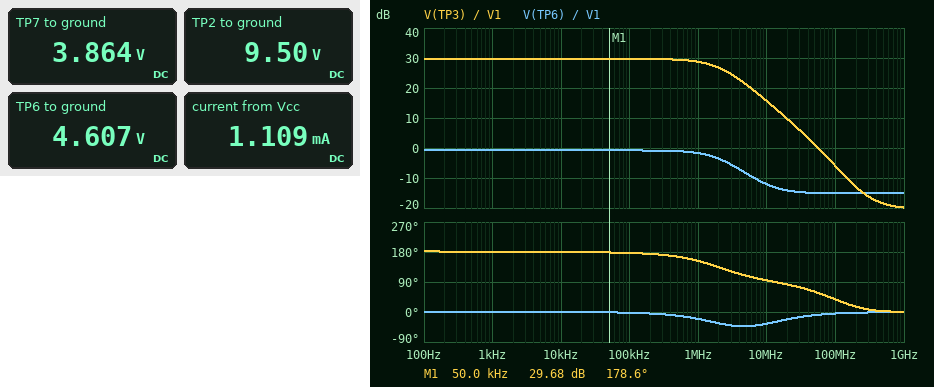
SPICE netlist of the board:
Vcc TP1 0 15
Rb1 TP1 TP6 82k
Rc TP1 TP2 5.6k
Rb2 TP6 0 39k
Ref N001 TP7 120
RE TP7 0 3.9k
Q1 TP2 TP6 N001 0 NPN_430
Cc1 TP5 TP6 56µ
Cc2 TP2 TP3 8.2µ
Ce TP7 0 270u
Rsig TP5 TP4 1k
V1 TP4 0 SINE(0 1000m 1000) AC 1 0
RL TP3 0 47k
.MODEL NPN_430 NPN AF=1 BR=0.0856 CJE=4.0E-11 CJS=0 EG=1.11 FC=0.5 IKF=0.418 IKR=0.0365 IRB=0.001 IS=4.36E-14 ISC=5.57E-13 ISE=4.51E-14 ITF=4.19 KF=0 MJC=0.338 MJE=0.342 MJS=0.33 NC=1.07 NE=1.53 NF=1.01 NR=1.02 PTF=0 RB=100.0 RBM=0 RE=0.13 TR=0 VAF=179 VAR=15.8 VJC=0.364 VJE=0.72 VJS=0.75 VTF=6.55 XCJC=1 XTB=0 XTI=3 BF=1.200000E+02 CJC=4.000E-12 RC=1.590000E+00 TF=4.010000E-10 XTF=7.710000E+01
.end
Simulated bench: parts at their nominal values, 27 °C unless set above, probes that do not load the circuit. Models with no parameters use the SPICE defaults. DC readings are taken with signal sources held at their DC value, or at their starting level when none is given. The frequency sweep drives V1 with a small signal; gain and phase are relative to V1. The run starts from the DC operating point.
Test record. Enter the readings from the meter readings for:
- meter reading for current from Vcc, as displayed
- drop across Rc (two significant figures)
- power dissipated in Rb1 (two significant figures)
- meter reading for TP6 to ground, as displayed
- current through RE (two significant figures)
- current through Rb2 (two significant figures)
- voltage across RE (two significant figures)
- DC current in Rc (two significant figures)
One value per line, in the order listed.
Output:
1.109 mA
5.5 V
1.3 mW
4.607 V
990 µA
120 µA
3.9 V
980 µA
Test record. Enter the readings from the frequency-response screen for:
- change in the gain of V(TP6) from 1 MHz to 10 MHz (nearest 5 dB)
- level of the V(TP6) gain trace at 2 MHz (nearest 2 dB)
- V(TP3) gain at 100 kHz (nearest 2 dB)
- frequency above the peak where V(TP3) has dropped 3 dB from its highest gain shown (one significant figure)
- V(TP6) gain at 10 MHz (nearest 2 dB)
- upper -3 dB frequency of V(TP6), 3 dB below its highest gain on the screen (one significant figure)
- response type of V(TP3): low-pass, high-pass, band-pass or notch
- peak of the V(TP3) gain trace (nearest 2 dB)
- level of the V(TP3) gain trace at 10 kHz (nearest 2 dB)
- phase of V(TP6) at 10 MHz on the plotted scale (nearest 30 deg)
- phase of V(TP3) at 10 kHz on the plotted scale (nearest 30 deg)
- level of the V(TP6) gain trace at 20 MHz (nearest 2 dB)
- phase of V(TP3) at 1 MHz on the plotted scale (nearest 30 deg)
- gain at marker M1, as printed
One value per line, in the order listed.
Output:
-10 dB
-4 dB
30 dB
2 MHz
-12 dB
2 MHz
low-pass
30 dB
30 dB
-30 deg
180 deg
-14 dB
150 deg
29.68 dB
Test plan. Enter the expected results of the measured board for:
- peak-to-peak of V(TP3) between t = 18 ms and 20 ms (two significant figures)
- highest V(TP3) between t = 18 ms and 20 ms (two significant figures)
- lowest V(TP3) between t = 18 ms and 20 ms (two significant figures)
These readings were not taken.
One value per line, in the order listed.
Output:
10 V
4.9 V
-5.2 V
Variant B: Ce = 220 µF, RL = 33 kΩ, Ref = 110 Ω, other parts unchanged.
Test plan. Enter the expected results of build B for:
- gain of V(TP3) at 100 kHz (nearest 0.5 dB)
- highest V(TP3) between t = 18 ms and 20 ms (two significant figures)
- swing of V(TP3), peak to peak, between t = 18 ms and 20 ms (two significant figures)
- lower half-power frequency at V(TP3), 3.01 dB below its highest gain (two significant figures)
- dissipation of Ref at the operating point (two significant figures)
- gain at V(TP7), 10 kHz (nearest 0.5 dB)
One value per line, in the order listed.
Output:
30.0 dB
4.7 V
9.9 V
5.3 Hz
110 µW
-66.5 dB
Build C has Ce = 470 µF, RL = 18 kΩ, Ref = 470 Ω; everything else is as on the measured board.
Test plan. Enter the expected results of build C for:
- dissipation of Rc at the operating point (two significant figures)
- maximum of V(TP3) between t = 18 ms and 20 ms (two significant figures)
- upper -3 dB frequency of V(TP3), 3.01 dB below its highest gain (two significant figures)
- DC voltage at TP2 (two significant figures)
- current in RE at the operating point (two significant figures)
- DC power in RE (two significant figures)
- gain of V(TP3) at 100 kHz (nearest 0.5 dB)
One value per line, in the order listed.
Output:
4.6 mW
3.9 V
5.8 MHz
9.9 V
920 µA
3.3 mW
18.0 dB
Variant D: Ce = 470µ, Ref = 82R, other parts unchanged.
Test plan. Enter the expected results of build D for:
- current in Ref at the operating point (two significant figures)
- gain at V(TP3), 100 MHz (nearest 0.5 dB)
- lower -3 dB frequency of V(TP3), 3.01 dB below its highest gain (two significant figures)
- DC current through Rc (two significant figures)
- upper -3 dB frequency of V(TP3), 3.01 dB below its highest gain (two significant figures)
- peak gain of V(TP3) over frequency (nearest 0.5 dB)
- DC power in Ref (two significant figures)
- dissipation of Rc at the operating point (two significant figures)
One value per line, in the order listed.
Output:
1.0 mA
-6.0 dB
3.2 Hz
990 µA
1.6 MHz
32.0 dB
82 µW
5.5 mW
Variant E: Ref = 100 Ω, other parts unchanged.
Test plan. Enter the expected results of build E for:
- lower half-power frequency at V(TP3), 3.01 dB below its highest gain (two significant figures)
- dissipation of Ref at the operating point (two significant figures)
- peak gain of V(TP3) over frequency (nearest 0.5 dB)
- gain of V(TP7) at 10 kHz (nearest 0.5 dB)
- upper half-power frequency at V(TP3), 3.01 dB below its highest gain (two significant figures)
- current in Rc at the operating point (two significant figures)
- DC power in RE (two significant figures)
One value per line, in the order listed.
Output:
4.7 Hz
99 µW
31.0 dB
-67.5 dB
1.8 MHz
990 µA
3.9 mW
